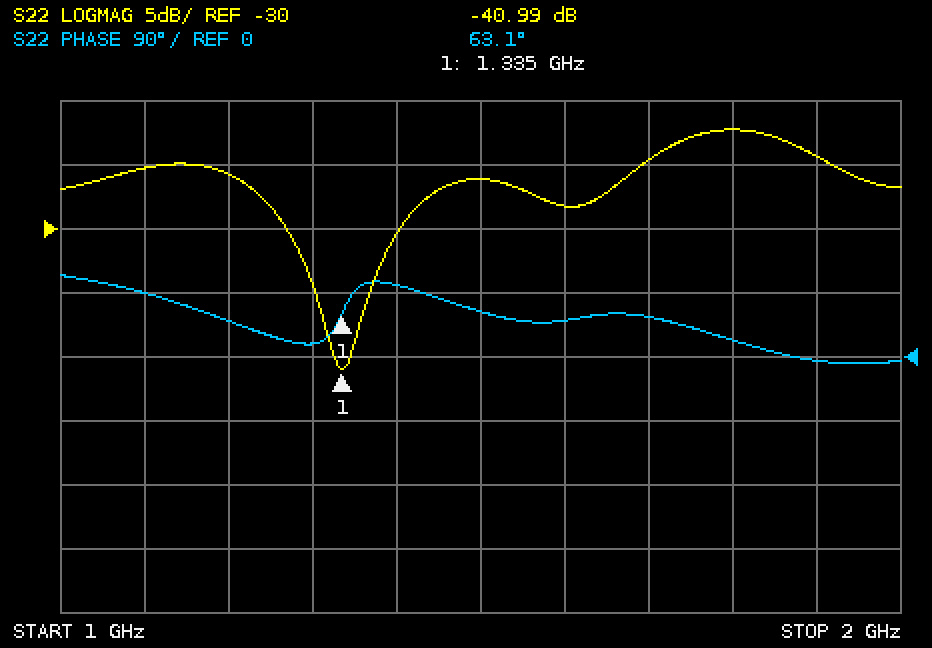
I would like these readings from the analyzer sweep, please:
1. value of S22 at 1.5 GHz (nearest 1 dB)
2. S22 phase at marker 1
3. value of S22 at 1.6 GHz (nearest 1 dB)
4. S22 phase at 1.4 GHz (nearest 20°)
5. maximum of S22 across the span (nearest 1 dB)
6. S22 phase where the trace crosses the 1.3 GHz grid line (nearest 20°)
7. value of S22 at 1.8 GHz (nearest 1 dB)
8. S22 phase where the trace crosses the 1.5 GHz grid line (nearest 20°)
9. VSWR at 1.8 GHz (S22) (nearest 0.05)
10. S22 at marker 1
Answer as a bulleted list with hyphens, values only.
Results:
- -26 dB
- 63.1°
- -28 dB
- 100°
- -22 dB
- 20°
- -22 dB
- 60°
- 1.15
- -40.99 dB
